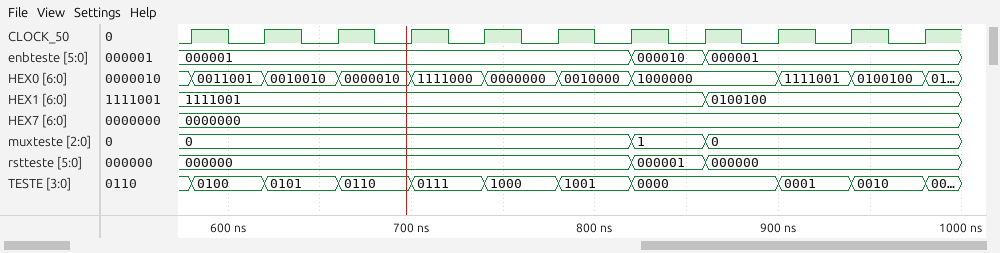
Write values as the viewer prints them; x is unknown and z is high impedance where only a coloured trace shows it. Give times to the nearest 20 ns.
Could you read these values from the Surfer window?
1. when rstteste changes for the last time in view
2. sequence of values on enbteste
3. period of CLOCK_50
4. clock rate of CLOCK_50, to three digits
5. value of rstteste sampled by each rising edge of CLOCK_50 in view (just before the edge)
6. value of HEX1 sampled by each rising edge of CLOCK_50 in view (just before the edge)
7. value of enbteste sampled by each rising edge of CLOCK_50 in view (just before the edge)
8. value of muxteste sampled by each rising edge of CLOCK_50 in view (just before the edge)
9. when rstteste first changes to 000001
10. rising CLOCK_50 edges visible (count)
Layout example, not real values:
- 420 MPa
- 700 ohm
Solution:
- 860 ns
- 000001, 000010, 000001
- 40 ns
- 25.0 MHz
- 000000, 000000, 000000, 000000, 000000, 000000, 000000, 000001, 000000, 000000, 000000
- 1111001, 1111001, 1111001, 1111001, 1111001, 1111001, 1111001, 1111001, 0100100, 0100100, 0100100
- 000001, 000001, 000001, 000001, 000001, 000001, 000001, 000010, 000001, 000001, 000001
- 0, 0, 0, 0, 0, 0, 0, 1, 0, 0, 0
- 820 ns
- 11
